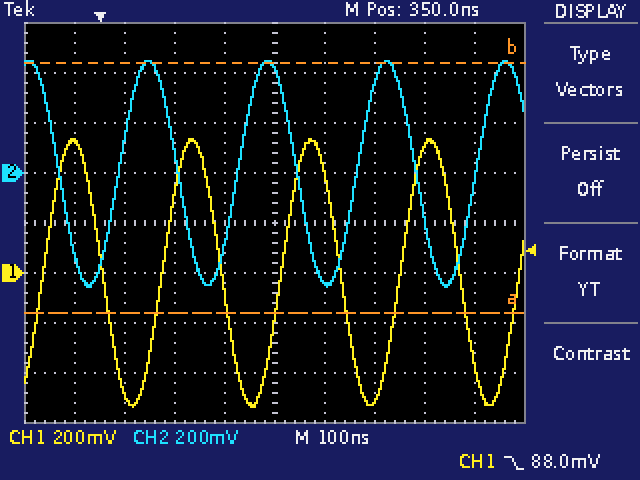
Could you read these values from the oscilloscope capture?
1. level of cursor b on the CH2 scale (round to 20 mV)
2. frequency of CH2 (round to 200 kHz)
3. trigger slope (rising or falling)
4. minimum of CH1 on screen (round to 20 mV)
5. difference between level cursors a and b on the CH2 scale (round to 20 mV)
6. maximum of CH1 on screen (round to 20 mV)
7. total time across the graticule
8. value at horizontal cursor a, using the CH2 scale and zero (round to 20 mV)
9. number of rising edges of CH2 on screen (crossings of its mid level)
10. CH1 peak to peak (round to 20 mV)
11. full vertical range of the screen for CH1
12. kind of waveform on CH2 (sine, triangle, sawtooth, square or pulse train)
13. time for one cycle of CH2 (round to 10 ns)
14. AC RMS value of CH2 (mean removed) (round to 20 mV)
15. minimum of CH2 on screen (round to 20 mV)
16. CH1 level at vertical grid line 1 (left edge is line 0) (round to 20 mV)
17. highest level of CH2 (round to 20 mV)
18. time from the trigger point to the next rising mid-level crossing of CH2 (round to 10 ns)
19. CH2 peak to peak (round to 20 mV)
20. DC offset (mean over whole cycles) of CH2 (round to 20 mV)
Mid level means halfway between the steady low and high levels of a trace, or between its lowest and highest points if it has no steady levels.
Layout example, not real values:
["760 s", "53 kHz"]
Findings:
["440 mV", "4.2 MHz", "falling", "-540 mV", "1.00 V", "540 mV", "1 µs", "-560 mV", "4", "1.08 V", "1.6 V", "sine", "240 ns", "320 mV", "-460 mV", "520 mV", "440 mV", "40 ns", "900 mV", "0 mV"]
